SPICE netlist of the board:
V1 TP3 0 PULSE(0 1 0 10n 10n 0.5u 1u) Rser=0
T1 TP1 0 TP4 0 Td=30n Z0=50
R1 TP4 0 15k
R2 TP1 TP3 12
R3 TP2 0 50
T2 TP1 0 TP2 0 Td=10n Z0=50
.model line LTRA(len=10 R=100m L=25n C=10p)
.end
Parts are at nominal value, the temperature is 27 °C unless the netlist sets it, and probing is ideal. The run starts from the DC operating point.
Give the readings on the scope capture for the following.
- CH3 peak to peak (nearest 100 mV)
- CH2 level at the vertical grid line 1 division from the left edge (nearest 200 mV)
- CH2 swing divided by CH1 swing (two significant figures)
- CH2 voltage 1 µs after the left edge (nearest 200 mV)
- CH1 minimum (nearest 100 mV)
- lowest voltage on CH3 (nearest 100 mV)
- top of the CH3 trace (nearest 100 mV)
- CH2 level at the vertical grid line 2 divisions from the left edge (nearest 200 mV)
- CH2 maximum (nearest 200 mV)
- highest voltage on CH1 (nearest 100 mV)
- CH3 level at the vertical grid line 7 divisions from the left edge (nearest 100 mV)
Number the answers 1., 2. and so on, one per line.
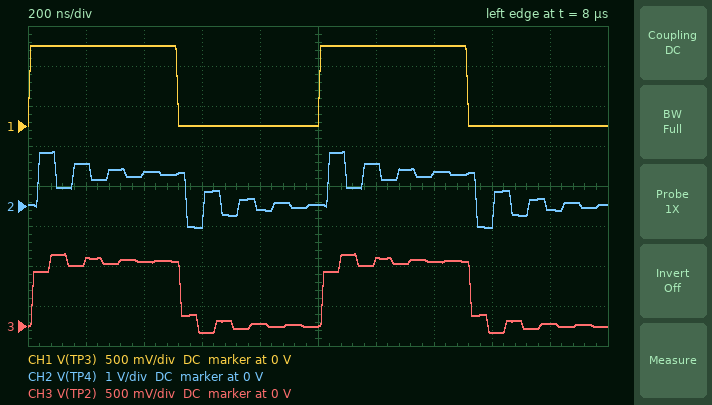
1. 1.0 V
2. 1.0 V
3. 1.9
4. 0 V
5. 0 V
6. -100 mV
7. 900 mV
8. 800 mV
9. 1.4 V
10. 1.0 V
11. 800 mV
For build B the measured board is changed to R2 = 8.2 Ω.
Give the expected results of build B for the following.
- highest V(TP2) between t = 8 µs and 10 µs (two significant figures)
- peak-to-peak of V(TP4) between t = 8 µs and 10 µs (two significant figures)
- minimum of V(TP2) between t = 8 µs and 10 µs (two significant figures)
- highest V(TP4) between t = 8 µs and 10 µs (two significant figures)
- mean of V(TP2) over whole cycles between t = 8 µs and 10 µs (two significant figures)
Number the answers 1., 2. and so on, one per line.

1. 940 mV
2. 2.2 V
3. -84 mV
4. 1.5 V
5. 440 mV
